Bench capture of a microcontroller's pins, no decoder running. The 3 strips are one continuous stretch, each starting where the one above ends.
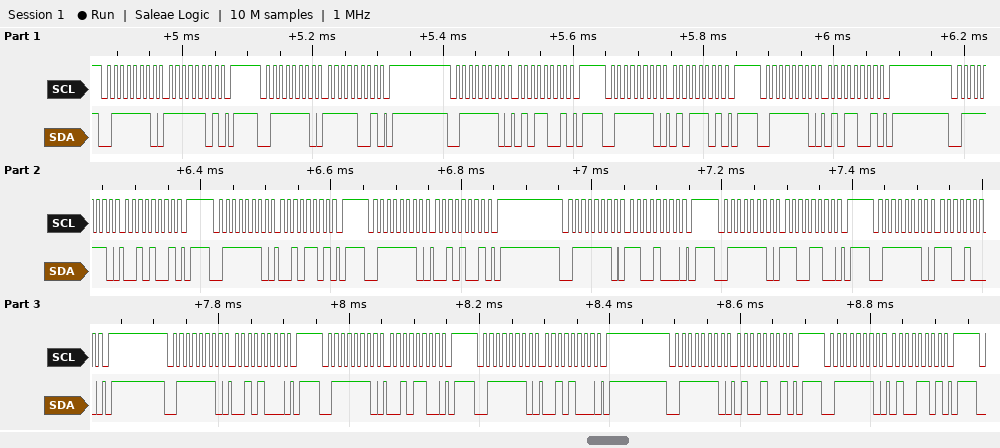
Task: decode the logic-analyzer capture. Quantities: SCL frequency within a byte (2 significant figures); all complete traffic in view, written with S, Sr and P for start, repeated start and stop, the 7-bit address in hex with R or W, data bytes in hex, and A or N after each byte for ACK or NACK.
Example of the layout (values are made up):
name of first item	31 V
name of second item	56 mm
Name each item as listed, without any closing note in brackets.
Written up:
SCL frequency within a byte	100 kHz
all complete traffic in view, written with S, Sr and P for start, repeated start and stop, the 7-bit address in hex with R or W, data bytes in hex, and A or N after each byte for ACK or NACK	S 3FW A FD A P S 3FW A F9 A P S 3FW A 59 A P S 3FW A 5D A P S 3FW A 59 A P S 3FW A 29 A P S 3FW A 2D A P S 3FW A 29 A P S 3FW A C8 A P S 3FW A CC A P S 3FW A C8 A P S 3FW A 28 A P S 3FW A 2C A P S 3FW A 28 A P S 3FW A 49 A P S 3FW A 4D A P
